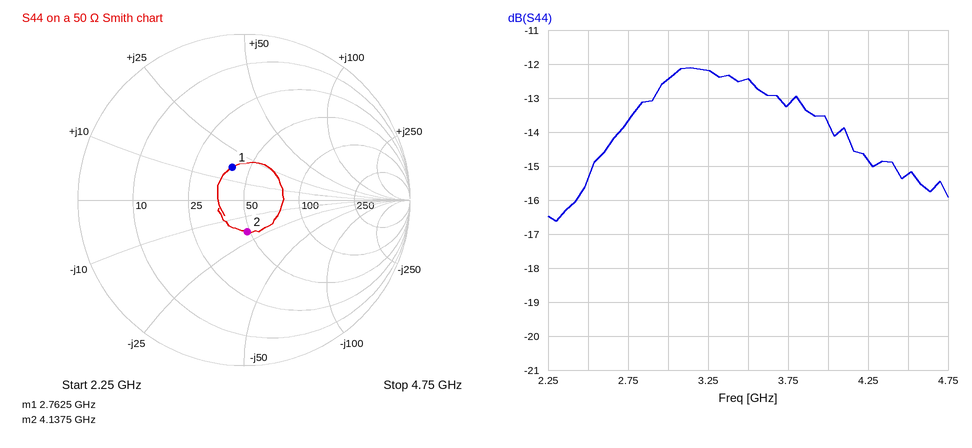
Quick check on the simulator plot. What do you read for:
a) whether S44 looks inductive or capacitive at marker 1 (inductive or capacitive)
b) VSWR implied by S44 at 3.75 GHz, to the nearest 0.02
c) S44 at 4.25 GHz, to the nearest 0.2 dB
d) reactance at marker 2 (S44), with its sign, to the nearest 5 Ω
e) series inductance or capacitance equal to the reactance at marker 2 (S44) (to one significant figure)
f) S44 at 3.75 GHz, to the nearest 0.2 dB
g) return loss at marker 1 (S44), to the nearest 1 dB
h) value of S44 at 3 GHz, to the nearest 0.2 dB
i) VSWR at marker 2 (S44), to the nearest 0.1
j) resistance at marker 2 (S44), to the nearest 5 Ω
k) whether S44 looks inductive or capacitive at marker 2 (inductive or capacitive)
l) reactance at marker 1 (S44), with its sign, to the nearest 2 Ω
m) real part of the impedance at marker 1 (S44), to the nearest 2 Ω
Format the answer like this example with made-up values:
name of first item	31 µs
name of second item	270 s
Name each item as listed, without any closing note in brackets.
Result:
whether S44 looks inductive or capacitive at marker 1	inductive
VSWR implied by S44 at 3.75 GHz, to the nearest 0.02	1.56
S44 at 4.25 GHz, to the nearest 0.2 dB	-14.8 dB
reactance at marker 2 (S44), with its sign, to the nearest 5 Ω	-20 Ω
series inductance or capacitance equal to the reactance at marker 2 (S44)	2 pF
S44 at 3.75 GHz, to the nearest 0.2 dB	-13.2 dB
return loss at marker 1 (S44), to the nearest 1 dB	14 dB
value of S44 at 3 GHz, to the nearest 0.2 dB	-12.4 dB
VSWR at marker 2 (S44), to the nearest 0.1	1.5
resistance at marker 2 (S44), to the nearest 5 Ω	50 Ω
whether S44 looks inductive or capacitive at marker 2	capacitive
reactance at marker 1 (S44), with its sign, to the nearest 2 Ω	+16 Ω
real part of the impedance at marker 1 (S44), to the nearest 2 Ω	40 Ω
